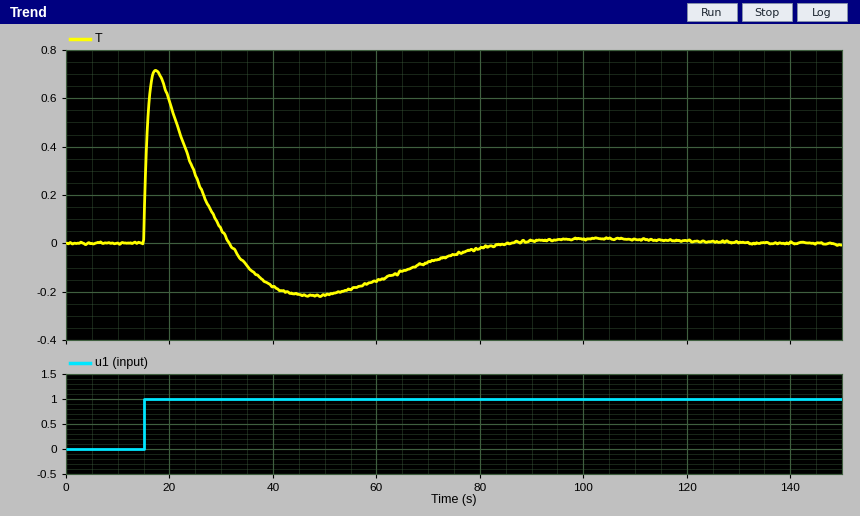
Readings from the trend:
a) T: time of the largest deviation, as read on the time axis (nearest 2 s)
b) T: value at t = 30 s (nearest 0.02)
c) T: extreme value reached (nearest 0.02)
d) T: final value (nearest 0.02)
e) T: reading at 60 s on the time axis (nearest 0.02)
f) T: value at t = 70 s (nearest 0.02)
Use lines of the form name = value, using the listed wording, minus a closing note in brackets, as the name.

T: time of the largest deviation, as read on the time axis = 18 s
T: value at t = 30 s = 0.06
T: extreme value reached = 0.72
T: final value = 0.00
T: reading at 60 s on the time axis = -0.16
T: value at t = 70 s = -0.08
